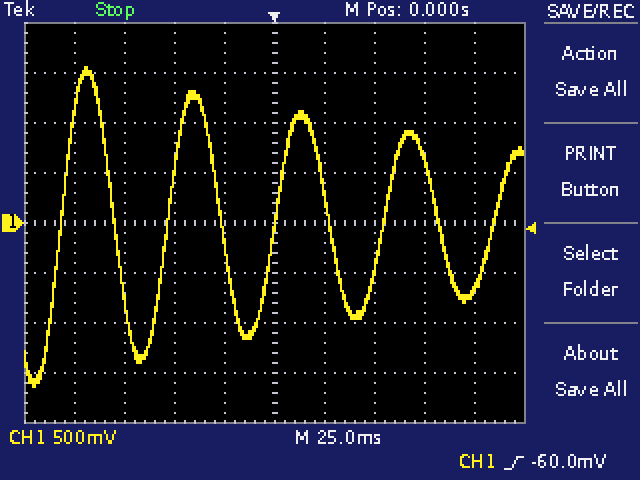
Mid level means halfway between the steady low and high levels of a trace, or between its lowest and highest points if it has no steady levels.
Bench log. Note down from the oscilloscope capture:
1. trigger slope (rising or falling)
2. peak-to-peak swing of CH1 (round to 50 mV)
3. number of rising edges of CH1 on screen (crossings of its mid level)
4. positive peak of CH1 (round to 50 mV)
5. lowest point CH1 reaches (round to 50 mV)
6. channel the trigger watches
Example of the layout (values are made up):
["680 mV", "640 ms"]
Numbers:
["rising", "3.20 V", "5", "1.55 V", "-1.65 V", "CH1"]
